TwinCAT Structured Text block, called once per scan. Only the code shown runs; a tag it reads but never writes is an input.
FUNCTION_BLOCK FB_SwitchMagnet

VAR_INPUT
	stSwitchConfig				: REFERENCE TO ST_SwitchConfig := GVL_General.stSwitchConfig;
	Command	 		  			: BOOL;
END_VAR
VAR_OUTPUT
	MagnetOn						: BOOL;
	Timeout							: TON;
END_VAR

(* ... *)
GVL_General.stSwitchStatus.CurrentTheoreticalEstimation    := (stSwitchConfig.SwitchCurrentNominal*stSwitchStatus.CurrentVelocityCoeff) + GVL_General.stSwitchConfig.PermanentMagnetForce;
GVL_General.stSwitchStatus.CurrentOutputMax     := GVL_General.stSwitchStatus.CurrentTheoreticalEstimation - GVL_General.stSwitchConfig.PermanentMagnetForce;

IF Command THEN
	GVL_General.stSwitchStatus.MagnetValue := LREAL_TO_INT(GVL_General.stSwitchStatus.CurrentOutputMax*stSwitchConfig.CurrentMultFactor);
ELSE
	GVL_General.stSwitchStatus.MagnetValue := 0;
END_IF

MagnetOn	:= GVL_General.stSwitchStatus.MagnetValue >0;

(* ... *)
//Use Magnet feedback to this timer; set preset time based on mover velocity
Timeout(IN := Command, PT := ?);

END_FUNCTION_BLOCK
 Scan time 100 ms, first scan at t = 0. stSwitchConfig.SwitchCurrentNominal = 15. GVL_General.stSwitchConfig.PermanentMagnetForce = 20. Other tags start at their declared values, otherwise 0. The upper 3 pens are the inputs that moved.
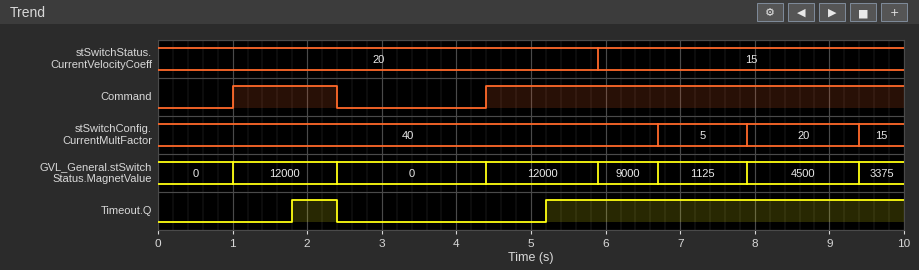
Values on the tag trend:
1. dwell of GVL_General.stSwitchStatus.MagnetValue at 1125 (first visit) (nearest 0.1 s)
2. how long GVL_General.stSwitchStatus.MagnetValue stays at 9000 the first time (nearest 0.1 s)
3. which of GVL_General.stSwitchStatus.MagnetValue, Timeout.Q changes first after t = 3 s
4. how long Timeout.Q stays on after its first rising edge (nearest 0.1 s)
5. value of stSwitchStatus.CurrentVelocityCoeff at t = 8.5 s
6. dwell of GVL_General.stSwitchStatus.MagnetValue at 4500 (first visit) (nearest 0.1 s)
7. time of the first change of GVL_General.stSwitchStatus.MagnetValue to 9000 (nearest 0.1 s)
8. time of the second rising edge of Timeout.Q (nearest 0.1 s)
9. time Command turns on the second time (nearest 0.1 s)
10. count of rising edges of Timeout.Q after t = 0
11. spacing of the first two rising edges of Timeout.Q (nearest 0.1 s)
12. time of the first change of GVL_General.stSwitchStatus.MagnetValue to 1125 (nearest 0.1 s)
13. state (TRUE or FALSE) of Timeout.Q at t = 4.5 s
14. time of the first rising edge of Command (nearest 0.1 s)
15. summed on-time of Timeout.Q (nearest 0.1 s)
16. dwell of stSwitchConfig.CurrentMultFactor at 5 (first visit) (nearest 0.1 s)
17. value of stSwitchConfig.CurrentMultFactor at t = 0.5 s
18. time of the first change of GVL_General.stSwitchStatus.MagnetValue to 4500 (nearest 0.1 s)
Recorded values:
1.2 s
0.8 s
GVL_General.stSwitchStatus.MagnetValue
0.6 s
15
1.5 s
5.9 s
5.2 s
4.4 s
2
3.4 s
6.7 s
FALSE
1.0 s
5.4 s
1.2 s
40
7.9 s
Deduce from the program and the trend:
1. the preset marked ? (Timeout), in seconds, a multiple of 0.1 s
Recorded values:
0.8 s
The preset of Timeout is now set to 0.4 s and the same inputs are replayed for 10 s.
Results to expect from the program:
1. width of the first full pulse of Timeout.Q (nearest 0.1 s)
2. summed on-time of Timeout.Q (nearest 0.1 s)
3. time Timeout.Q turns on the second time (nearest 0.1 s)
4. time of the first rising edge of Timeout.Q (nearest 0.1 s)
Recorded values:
1.0 s
6.2 s
4.8 s
1.4 s
